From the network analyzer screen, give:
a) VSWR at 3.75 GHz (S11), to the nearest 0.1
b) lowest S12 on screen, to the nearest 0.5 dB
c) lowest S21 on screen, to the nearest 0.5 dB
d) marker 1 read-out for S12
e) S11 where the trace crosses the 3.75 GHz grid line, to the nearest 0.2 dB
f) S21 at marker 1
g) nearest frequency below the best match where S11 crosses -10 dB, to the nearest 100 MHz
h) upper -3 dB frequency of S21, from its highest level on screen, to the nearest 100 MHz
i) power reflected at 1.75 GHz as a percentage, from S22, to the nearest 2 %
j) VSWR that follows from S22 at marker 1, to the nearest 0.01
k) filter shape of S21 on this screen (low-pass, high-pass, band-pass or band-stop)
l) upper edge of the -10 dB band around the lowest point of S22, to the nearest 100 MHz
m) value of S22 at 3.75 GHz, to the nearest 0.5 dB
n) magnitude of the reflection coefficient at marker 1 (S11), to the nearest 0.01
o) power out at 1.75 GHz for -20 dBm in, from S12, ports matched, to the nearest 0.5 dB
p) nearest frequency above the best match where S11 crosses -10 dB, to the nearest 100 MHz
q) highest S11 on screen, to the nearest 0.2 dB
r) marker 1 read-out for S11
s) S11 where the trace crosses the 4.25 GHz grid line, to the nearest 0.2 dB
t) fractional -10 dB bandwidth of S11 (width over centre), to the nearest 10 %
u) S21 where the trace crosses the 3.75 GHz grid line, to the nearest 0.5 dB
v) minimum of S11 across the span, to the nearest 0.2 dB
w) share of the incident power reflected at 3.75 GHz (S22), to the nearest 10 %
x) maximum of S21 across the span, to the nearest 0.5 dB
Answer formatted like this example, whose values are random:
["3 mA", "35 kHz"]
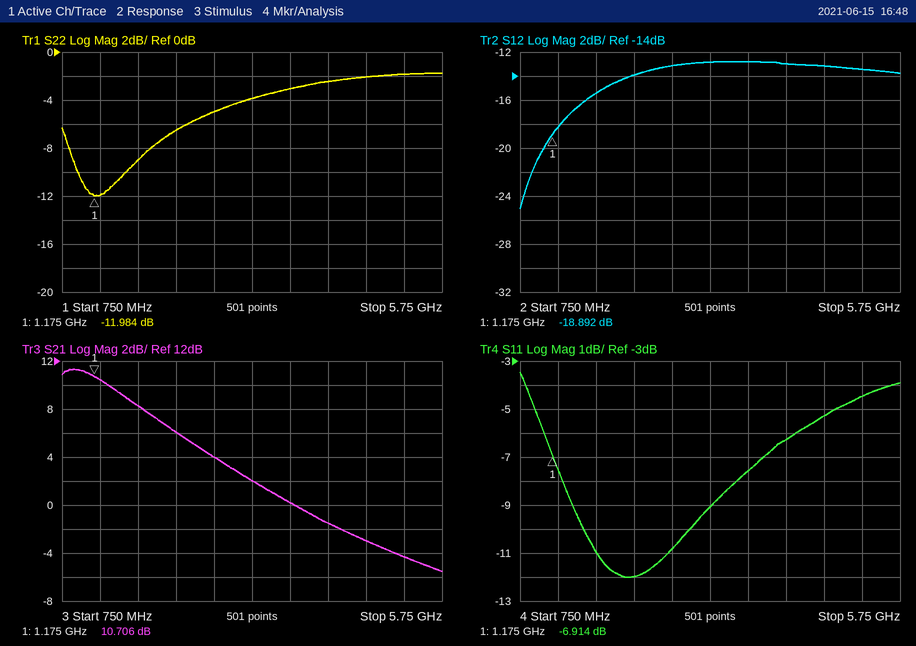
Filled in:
["2.4", "-25.0 dB", "-5.5 dB", "-18.892 dB", "-7.6 dB", "10.706 dB", "1.6 GHz", "1.7 GHz", "12 %", "1.67", "low-pass", "1.6 GHz", "-3.0 dB", "0.45", "-35.5 dBm", "3.0 GHz", "-3.4 dB", "-6.914 dB", "-6.2 dB", "60 %", "0.0 dB", "-12.0 dB", "50 %", "11.5 dB"]
